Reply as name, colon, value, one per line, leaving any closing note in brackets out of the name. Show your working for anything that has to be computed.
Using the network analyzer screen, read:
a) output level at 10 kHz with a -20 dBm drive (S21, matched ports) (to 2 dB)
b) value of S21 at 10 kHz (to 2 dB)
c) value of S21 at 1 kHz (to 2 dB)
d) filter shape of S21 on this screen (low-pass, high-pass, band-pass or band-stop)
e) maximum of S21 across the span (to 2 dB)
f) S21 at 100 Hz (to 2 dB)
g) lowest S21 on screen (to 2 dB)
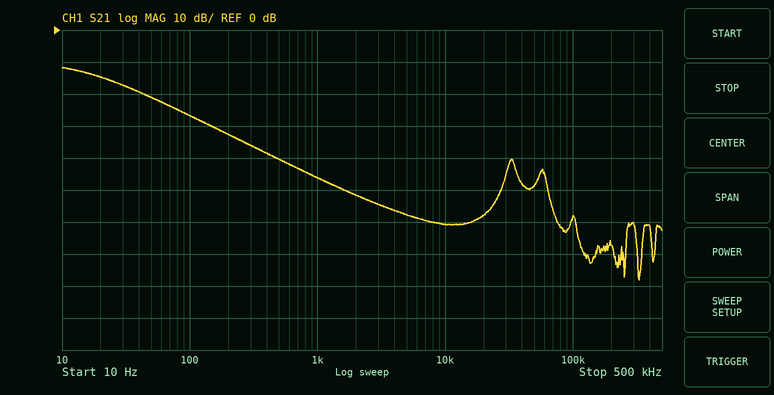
output level at 10 kHz with a -20 dBm drive (S21, matched ports): -20 dBm + (-60 dB) = -80 dBm
value of S21 at 10 kHz: -60 dB
value of S21 at 1 kHz: -46 dB
filter shape of S21 on this screen: low-pass
maximum of S21 across the span: -12 dB
S21 at 100 Hz: -26 dB
lowest S21 on screen: -78 dB
